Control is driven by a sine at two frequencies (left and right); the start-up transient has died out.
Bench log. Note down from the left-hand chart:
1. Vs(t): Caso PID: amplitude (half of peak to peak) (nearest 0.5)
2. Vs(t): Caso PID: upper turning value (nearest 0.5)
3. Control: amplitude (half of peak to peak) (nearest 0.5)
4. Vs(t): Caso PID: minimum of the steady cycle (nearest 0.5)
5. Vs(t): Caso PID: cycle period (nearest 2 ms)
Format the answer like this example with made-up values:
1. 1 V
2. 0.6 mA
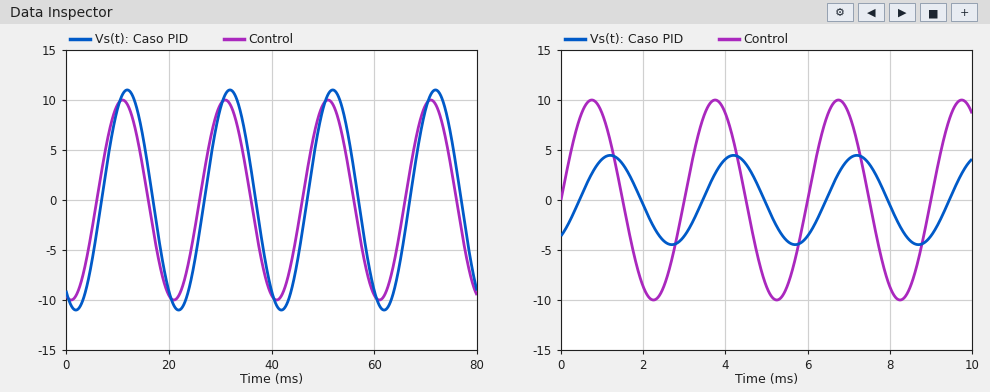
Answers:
1. 11.0
2. 11.0
3. 10.0
4. -11.0
5. 20 ms
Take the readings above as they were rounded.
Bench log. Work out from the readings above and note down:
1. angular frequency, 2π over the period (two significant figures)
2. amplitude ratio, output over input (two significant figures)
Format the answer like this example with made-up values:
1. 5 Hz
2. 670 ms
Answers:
1. 0.31 rad/ms
2. 1.1
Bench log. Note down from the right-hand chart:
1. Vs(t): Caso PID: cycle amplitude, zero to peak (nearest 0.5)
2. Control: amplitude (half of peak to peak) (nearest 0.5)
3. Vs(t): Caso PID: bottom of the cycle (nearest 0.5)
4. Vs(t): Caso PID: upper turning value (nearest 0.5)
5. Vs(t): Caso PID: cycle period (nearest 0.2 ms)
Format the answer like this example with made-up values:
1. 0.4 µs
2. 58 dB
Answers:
1. 4.5
2. 10.0
3. -4.5
4. 4.5
5. 3.0 ms
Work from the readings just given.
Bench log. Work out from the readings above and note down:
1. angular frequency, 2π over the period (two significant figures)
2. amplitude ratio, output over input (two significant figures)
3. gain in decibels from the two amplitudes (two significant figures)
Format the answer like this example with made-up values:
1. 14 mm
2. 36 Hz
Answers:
1. 2.1 rad/ms
2. 0.45
3. -6.9 dB
